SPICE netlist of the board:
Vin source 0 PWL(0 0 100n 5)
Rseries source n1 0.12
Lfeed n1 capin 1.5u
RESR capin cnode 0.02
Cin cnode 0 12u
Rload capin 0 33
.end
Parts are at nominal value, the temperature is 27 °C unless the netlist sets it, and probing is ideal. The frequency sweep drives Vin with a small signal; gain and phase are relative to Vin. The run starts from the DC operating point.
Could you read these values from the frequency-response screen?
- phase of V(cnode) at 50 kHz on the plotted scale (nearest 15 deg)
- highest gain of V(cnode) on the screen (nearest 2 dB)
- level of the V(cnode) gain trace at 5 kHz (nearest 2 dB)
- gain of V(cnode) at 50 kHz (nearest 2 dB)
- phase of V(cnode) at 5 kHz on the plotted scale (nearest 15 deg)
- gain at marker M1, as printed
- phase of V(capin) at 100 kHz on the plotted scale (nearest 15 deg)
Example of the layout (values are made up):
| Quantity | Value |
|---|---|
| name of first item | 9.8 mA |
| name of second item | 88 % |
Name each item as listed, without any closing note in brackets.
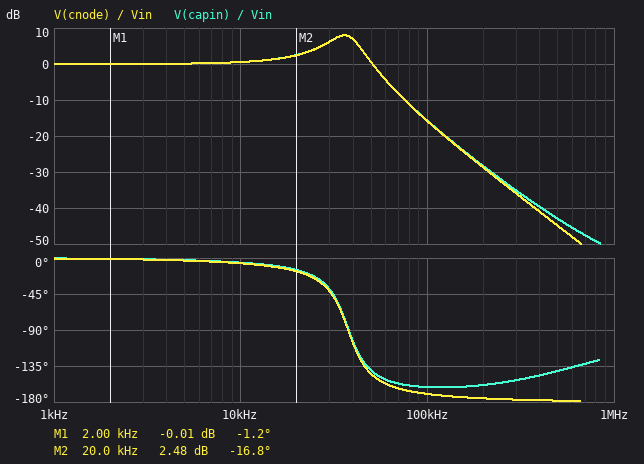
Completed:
| Quantity | Value |
|---|---|
| phase of V(cnode) at 50 kHz on the plotted scale | -150 deg |
| highest gain of V(cnode) on the screen | 8 dB |
| level of the V(cnode) gain trace at 5 kHz | 0 dB |
| gain of V(cnode) at 50 kHz | 0 dB |
| phase of V(cnode) at 5 kHz on the plotted scale | 0 deg |
| gain at marker M1, as printed | -0.01 dB |
| phase of V(capin) at 100 kHz on the plotted scale | -165 deg |
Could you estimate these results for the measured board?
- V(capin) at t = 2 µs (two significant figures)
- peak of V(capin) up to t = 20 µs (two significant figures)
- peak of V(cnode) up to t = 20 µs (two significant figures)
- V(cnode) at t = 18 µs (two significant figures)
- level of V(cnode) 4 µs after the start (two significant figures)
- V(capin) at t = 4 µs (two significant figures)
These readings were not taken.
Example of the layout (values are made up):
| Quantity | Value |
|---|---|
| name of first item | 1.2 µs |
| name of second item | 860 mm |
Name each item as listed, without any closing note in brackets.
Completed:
| Quantity | Value |
|---|---|
| V(capin) at t = 2 µs | 600 mV |
| peak of V(capin) up to t = 20 µs | 7.6 V |
| peak of V(cnode) up to t = 20 µs | 7.6 V |
| V(cnode) at t = 18 µs | 6.5 V |
| level of V(cnode) 4 µs after the start | 1.8 V |
| V(capin) at t = 4 µs | 2.0 V |
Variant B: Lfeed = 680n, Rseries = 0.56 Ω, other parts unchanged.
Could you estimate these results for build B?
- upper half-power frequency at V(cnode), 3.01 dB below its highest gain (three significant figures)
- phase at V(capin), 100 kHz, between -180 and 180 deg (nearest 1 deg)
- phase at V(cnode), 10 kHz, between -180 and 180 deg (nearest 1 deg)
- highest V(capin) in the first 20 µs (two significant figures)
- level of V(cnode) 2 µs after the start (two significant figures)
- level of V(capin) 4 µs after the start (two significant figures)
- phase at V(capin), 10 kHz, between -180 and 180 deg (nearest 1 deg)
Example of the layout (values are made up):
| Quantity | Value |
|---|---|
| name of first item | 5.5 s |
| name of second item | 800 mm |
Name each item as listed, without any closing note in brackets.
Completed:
| Quantity | Value |
|---|---|
| upper half-power frequency at V(cnode), 3.01 dB below its highest gain | 27.7 kHz |
| phase at V(capin), 100 kHz, between -180 and 180 deg | -108 deg |
| phase at V(cnode), 10 kHz, between -180 and 180 deg | -24 deg |
| highest V(capin) in the first 20 µs | 4.8 V |
| level of V(cnode) 2 µs after the start | 690 mV |
| level of V(capin) 4 µs after the start | 1.9 V |
| phase at V(capin), 10 kHz, between -180 and 180 deg | -23 deg |
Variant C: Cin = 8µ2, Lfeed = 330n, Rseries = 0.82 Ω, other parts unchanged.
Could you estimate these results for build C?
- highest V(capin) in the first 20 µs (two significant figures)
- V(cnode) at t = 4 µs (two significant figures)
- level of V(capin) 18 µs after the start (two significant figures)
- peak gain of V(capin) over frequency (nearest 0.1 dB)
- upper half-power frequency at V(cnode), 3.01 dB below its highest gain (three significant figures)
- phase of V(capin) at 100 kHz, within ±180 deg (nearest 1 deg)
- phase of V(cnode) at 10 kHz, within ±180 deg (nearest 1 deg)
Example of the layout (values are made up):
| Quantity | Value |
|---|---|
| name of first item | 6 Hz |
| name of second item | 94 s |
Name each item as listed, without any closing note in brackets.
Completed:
| Quantity | Value |
|---|---|
| highest V(capin) in the first 20 µs | 4.7 V |
| V(cnode) at t = 4 µs | 2.1 V |
| level of V(capin) 18 µs after the start | 4.6 V |
| peak gain of V(capin) over frequency | -0.2 dB |
| upper half-power frequency at V(cnode), 3.01 dB below its highest gain | 25.1 kHz |
| phase of V(capin) at 100 kHz, within ±180 deg | -85 deg |
| phase of V(cnode) at 10 kHz, within ±180 deg | -23 deg |
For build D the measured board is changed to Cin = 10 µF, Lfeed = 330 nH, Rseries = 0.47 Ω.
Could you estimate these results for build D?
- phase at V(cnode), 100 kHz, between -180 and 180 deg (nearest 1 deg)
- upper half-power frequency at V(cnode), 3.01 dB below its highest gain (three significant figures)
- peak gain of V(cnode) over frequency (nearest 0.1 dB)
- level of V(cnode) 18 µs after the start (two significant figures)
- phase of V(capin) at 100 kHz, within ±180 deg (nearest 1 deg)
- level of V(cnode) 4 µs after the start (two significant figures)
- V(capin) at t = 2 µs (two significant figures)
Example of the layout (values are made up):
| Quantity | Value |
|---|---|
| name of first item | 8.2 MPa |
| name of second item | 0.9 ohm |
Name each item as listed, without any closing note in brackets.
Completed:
| Quantity | Value |
|---|---|
| phase at V(cnode), 100 kHz, between -180 and 180 deg | -95 deg |
| upper half-power frequency at V(cnode), 3.01 dB below its highest gain | 38.0 kHz |
| peak gain of V(cnode) over frequency | -0.1 dB |
| level of V(cnode) 18 µs after the start | 4.9 V |
| phase of V(capin) at 100 kHz, within ±180 deg | -88 deg |
| level of V(cnode) 4 µs after the start | 2.6 V |
| V(capin) at t = 2 µs | 1.4 V |
